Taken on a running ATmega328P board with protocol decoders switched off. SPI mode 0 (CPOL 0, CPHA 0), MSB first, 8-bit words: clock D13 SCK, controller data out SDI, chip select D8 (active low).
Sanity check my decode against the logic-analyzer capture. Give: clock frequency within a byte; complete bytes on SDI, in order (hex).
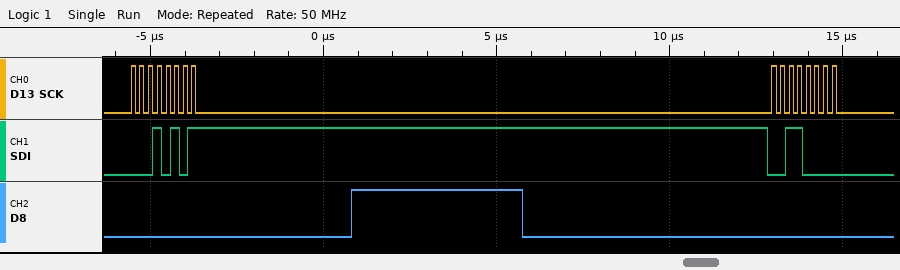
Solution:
4 MHz
15 30
